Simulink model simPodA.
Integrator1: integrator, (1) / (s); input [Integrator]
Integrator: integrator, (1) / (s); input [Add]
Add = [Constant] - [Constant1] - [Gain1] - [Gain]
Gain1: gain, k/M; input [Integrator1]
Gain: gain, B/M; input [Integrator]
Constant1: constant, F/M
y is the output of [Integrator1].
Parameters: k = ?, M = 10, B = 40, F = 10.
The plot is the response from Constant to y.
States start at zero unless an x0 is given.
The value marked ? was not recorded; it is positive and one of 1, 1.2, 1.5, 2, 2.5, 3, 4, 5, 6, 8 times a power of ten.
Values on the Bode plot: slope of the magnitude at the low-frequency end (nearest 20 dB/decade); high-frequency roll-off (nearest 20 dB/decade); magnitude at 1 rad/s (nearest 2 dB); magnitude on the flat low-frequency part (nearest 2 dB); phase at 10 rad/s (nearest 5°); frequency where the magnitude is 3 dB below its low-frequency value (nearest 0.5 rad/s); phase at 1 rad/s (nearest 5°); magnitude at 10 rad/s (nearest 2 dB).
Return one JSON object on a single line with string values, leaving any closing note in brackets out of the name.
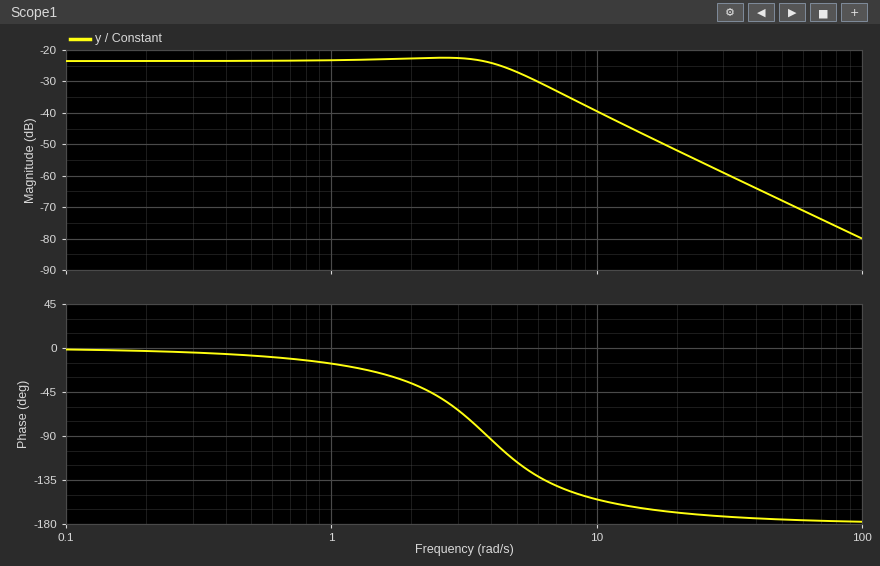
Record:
{"slope of the magnitude at the low-frequency end": "0 dB/decade", "high-frequency roll-off": "-40 dB/decade", "magnitude at 1 rad/s": "-24 dB", "magnitude on the flat low-frequency part": "-24 dB", "phase at 10 rad/s": "-155°", "frequency where the magnitude is 3 dB below its low-frequency value": "5.0 rad/s", "phase at 1 rad/s": "-15°", "magnitude at 10 rad/s": "-40 dB"}
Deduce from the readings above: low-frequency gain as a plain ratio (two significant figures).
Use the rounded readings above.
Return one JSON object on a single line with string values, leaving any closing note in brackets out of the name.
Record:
{"low-frequency gain as a plain ratio": "0.063"}
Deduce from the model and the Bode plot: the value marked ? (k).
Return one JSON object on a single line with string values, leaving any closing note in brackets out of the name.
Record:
{"the value marked ?": "150"}
